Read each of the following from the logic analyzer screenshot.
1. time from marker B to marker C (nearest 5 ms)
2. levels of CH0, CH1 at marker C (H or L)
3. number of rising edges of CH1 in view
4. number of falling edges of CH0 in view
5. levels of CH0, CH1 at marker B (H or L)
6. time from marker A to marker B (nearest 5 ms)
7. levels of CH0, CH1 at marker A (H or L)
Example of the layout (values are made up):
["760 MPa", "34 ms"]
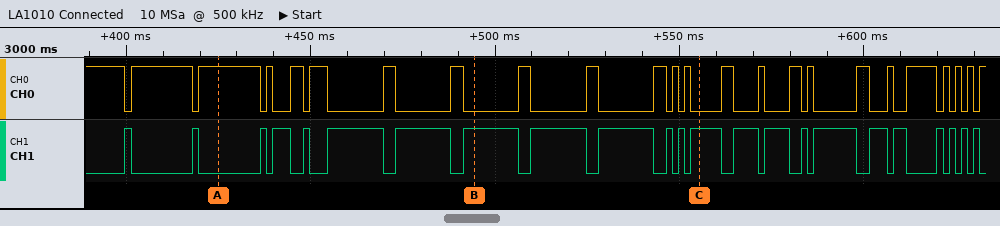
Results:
["60 ms", "CH0=L, CH1=H", "23", "23", "CH0=L, CH1=H", "70 ms", "CH0=H, CH1=L"]
